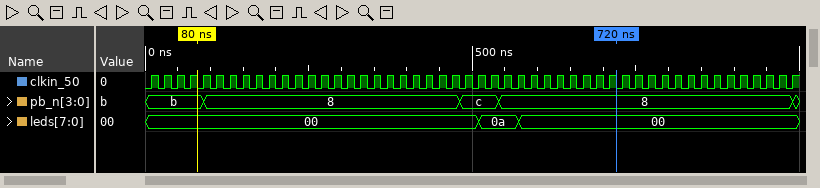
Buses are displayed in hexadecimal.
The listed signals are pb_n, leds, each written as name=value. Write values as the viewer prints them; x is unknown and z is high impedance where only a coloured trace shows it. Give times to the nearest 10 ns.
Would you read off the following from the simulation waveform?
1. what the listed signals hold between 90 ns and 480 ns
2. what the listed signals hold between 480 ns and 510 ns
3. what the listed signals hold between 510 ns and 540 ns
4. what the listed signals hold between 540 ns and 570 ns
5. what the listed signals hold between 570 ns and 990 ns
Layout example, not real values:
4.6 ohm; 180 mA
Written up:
pb_n=8, leds=00; pb_n=c, leds=00; pb_n=c, leds=0a; pb_n=8, leds=0a; pb_n=8, leds=00
